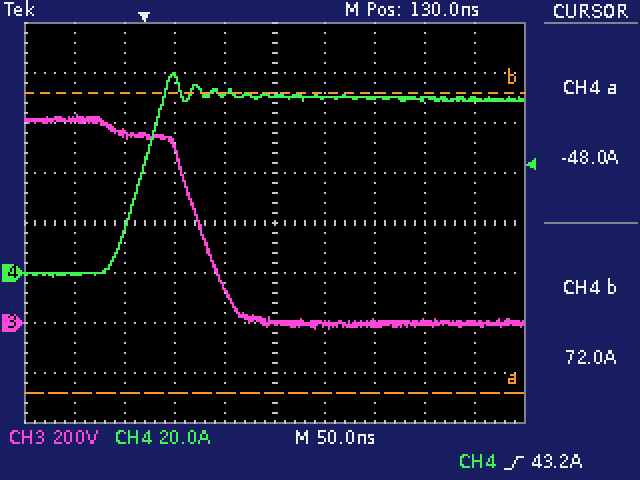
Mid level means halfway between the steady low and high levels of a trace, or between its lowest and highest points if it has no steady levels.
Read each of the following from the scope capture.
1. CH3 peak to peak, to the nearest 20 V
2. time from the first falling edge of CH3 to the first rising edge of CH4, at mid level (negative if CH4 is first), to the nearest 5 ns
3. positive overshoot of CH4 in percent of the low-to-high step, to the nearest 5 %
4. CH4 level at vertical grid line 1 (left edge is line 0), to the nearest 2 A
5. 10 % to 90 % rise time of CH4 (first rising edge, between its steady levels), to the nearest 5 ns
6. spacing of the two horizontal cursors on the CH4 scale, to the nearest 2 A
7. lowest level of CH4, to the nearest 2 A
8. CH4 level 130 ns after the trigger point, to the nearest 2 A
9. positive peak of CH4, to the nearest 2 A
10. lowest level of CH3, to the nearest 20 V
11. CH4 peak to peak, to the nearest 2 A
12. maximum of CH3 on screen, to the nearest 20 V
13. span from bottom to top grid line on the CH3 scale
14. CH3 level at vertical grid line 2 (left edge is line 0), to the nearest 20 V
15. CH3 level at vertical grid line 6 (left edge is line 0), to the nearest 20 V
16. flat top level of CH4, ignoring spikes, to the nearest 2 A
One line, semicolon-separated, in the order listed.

860 V; -60 ns; 15 %; 0 A; 45 ns; 120 A; -2 A; 70 A; 80 A; -20 V; 82 A; 840 V; 1.6 kV; 760 V; 0 V; 70 A
